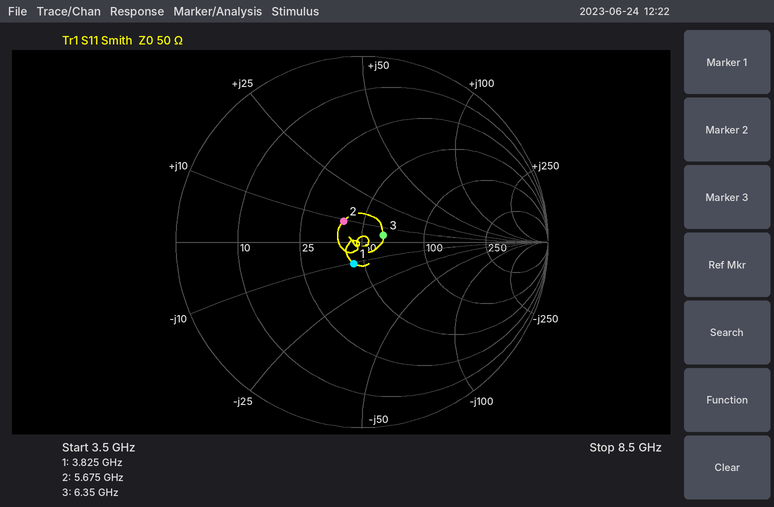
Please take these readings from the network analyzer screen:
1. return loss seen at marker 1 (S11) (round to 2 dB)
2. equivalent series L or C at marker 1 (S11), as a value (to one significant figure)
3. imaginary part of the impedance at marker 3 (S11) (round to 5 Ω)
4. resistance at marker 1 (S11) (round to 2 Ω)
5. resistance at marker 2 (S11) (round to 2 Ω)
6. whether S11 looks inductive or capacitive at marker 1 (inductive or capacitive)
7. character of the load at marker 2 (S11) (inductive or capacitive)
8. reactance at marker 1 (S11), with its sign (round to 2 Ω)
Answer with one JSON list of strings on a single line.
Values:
["18 dB", "4 pF", "+5 Ω", "44 Ω", "40 Ω", "capacitive", "inductive", "-10 Ω"]
